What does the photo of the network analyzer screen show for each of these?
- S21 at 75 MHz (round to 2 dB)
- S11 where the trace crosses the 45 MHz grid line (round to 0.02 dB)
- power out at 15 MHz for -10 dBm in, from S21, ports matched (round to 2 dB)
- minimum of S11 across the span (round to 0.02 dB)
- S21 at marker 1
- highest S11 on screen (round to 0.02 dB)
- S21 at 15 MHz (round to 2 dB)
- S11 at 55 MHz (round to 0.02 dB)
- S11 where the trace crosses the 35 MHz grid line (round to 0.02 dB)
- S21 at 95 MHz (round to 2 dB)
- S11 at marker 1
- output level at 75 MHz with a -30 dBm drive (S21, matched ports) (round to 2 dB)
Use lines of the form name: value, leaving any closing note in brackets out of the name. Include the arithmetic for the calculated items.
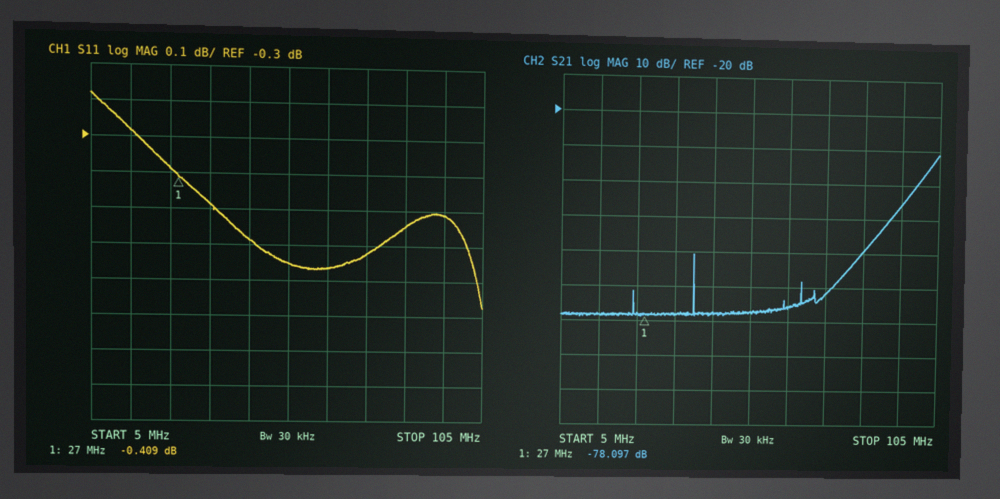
S21 at 75 MHz: -72 dB
S11 where the trace crosses the 45 MHz grid line: -0.58 dB
power out at 15 MHz for -10 dBm in, from S21, ports matched: -10 dBm + (-78 dB) = -88 dBm
minimum of S11 across the span: -0.78 dB
S21 at marker 1: -78.097 dB
highest S11 on screen: -0.18 dB
S21 at 15 MHz: -78 dB
S11 at 55 MHz: -0.66 dB
S11 where the trace crosses the 35 MHz grid line: -0.48 dB
S21 at 95 MHz: -46 dB
S11 at marker 1: -0.409 dB
output level at 75 MHz with a -30 dBm drive (S21, matched ports): -30 dBm + (-72 dB) = -102 dBm
